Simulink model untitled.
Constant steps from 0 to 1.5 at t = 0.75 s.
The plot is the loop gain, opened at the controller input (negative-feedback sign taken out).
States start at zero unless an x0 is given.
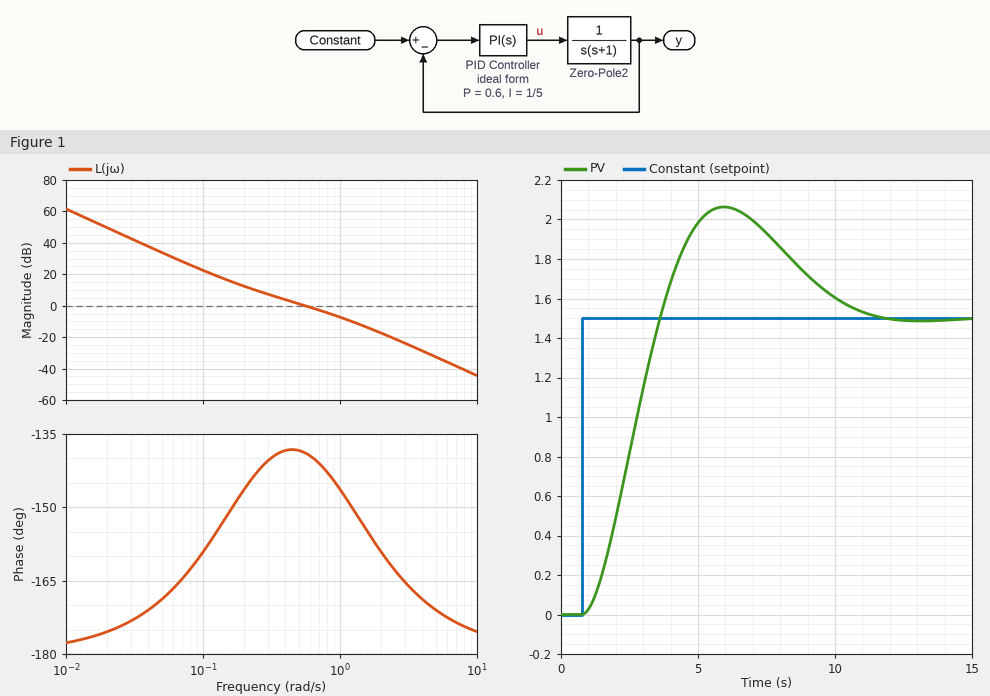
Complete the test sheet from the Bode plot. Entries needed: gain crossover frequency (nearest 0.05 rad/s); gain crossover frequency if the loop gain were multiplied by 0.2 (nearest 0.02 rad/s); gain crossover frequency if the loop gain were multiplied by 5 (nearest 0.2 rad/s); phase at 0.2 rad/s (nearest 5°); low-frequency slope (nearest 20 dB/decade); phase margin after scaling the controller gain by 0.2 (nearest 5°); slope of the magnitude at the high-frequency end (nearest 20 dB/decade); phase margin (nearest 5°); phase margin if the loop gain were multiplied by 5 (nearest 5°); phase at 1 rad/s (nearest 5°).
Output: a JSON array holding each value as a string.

["0.55 rad/s", "0.18 rad/s", "1.6 rad/s", "-145°", "-40 dB/decade", "30°", "-40 dB/decade", "40°", "25°", "-145°"]
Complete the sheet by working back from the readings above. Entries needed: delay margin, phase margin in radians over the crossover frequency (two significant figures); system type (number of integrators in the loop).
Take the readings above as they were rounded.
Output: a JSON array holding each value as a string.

["1.3 s", "2"]
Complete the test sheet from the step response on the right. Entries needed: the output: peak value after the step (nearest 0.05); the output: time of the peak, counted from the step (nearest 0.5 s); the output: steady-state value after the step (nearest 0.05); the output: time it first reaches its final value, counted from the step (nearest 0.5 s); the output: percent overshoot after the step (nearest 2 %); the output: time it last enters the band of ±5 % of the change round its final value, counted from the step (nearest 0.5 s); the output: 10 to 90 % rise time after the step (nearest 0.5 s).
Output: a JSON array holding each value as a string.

["2.05", "5.0 s", "1.50", "3.0 s", "38 %", "9.5 s", "2.0 s"]
